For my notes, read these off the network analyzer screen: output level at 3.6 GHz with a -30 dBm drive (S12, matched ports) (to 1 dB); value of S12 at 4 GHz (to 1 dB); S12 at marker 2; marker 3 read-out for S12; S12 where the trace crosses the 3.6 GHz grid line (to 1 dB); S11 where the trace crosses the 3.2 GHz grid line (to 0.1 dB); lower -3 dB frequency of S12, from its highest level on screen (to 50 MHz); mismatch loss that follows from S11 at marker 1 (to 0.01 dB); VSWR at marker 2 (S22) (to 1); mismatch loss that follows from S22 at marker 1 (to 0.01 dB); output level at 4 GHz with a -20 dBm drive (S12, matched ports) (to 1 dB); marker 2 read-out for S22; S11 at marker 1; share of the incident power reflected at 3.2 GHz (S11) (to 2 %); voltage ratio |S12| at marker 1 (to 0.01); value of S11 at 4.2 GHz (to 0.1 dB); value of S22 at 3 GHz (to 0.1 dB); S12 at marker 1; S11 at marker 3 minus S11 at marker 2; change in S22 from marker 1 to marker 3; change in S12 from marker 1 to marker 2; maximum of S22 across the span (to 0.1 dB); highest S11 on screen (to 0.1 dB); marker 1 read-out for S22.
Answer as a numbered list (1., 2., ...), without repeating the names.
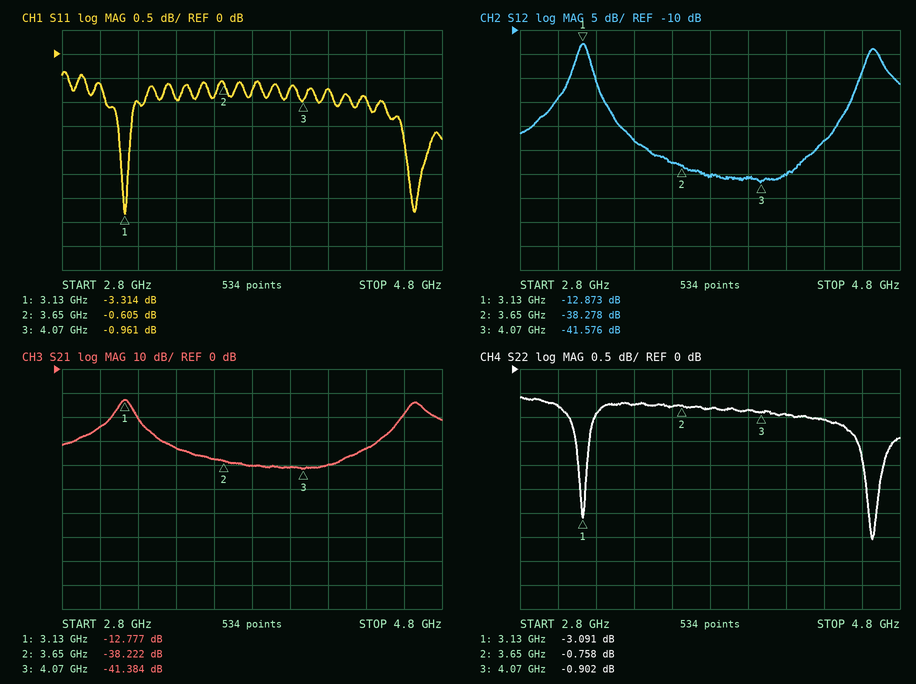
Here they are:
1. -68 dBm
2. -41 dB
3. -38.278 dB
4. -41.576 dB
5. -38 dB
6. -1.0 dB
7. 3.10 GHz
8. 2.73 dB
9. 23
10. 2.93 dB
11. -61 dBm
12. -0.758 dB
13. -3.314 dB
14. 80 %
15. 0.23
16. -0.7 dB
17. -0.8 dB
18. -12.873 dB
19. -0.356 dB
20. 2.189 dB
21. -25.405 dB
22. -0.6 dB
23. -0.4 dB
24. -3.091 dB
